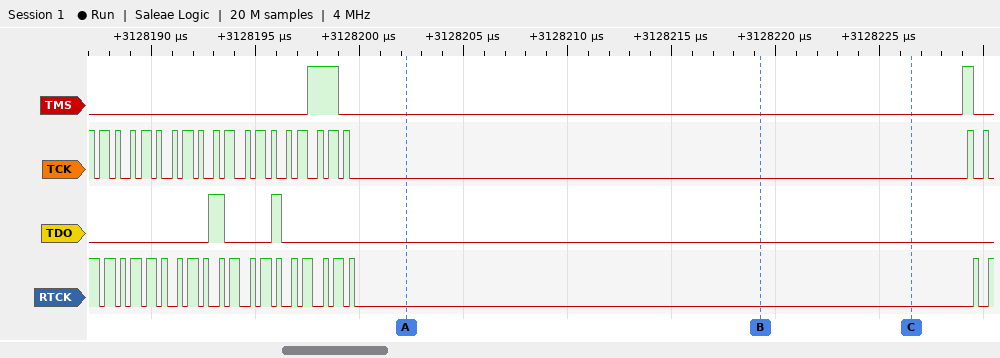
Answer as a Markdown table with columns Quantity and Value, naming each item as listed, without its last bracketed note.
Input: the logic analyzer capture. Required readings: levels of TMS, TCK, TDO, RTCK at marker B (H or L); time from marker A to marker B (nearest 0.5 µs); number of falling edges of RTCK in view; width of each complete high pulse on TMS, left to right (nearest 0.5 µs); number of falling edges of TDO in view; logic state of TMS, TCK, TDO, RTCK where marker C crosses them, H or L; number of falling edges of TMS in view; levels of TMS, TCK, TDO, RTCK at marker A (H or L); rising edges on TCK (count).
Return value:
| Quantity | Value |
|---|---|
| levels of TMS, TCK, TDO, RTCK at marker B | TMS=L, TCK=L, TDO=L, RTCK=L |
| time from marker A to marker B | 17 µs |
| number of falling edges of RTCK in view | 20 |
| width of each complete high pulse on TMS, left to right | 1.5 µs, 0.5 µs |
| number of falling edges of TDO in view | 2 |
| logic state of TMS, TCK, TDO, RTCK where marker C crosses them, H or L | TMS=L, TCK=L, TDO=L, RTCK=L |
| number of falling edges of TMS in view | 2 |
| levels of TMS, TCK, TDO, RTCK at marker A | TMS=L, TCK=L, TDO=L, RTCK=L |
| rising edges on TCK | 20 |
